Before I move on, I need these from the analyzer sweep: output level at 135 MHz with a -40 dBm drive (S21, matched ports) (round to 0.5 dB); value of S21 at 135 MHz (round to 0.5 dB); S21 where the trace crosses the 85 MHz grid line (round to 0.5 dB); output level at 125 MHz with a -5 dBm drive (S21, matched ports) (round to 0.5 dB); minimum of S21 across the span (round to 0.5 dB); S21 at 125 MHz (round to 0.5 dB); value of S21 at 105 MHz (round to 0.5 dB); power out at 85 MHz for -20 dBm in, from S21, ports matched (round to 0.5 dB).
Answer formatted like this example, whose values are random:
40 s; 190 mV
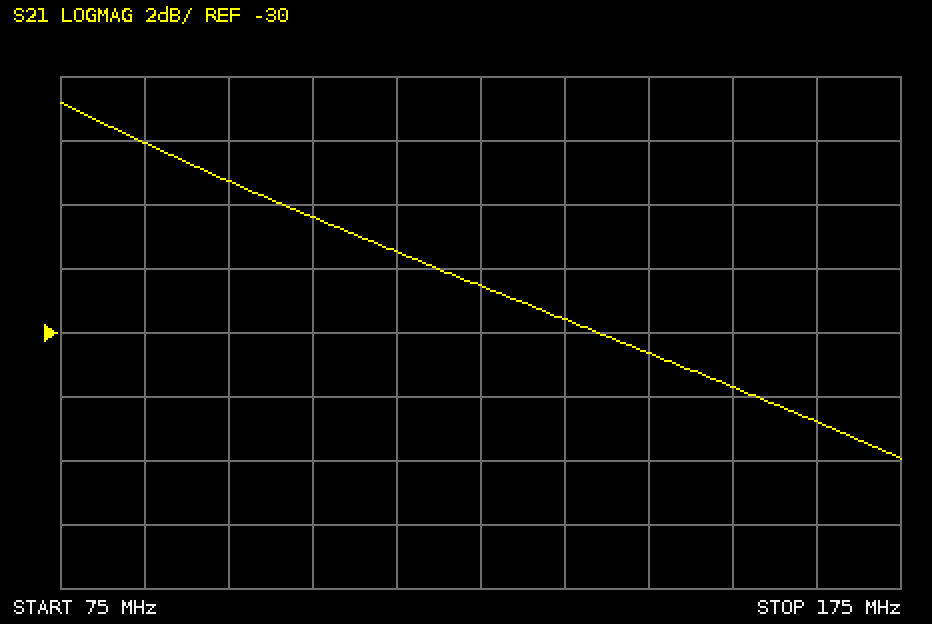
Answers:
-69.5 dBm; -29.5 dB; -24.0 dB; -33.5 dBm; -34.0 dB; -28.5 dB; -26.5 dB; -44.0 dBm
